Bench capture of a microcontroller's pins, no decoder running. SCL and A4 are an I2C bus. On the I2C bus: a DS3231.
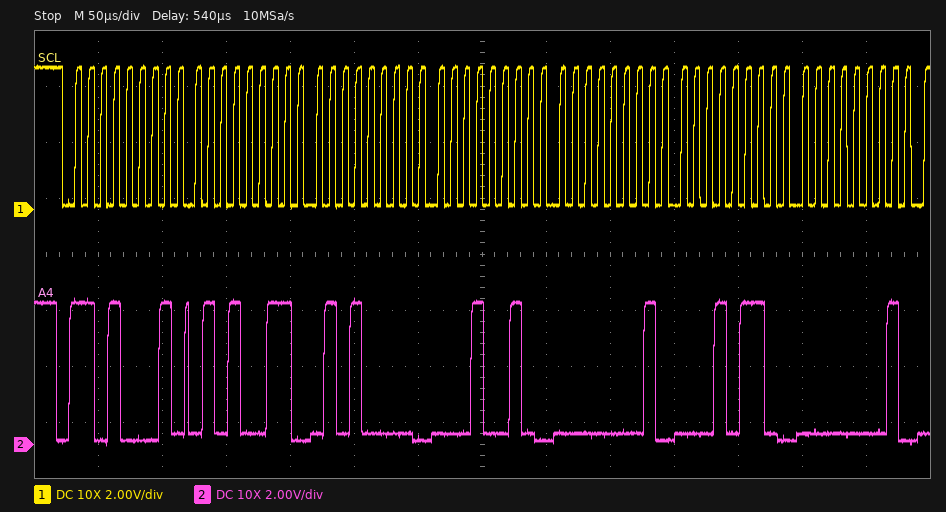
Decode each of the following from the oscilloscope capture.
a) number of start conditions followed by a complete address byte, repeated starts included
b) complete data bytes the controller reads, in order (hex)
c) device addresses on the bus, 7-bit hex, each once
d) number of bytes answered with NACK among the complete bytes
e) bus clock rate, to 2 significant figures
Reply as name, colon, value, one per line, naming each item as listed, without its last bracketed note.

number of start conditions followed by a complete address byte, repeated starts included: 1
complete data bytes the controller reads, in order: 53 50 12 01 16 01
device addresses on the bus, 7-bit hex, each once: 0x68
number of bytes answered with NACK among the complete bytes: 0
bus clock rate, to 2 significant figures: 100 kHz
